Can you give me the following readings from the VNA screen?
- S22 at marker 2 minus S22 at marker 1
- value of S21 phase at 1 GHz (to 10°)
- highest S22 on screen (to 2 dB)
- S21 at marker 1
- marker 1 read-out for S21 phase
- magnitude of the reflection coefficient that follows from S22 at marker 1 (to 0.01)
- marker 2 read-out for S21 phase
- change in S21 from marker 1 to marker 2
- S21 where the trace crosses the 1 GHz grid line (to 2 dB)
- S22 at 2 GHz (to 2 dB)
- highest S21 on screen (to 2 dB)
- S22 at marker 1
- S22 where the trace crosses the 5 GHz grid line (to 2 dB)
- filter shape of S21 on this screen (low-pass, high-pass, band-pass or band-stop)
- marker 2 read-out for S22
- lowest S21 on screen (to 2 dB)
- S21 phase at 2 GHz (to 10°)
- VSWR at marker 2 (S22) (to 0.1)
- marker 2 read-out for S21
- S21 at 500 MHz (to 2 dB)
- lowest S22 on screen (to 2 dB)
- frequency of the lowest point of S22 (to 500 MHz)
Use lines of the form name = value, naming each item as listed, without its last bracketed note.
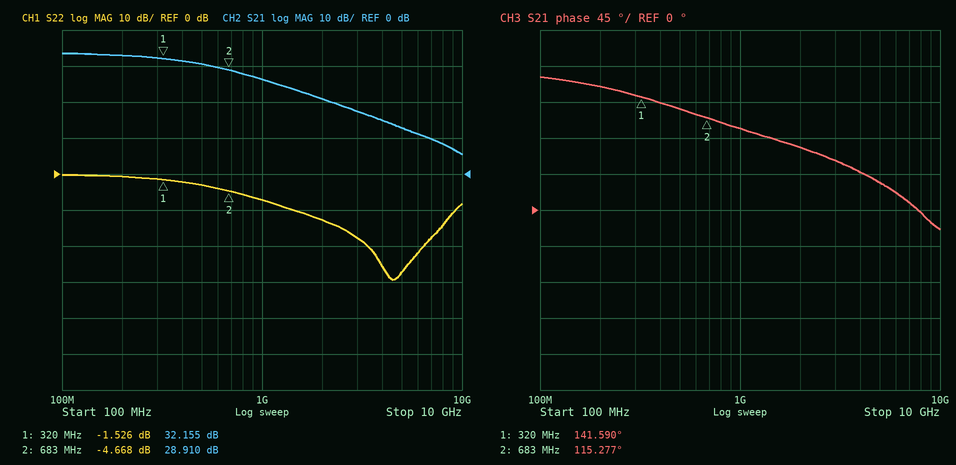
S22 at marker 2 minus S22 at marker 1 = -3.142 dB
value of S21 phase at 1 GHz = 100°
highest S22 on screen = 0 dB
S21 at marker 1 = 32.155 dB
marker 1 read-out for S21 phase = 141.590°
magnitude of the reflection coefficient that follows from S22 at marker 1 = 0.84
marker 2 read-out for S21 phase = 115.277°
change in S21 from marker 1 to marker 2 = -3.245 dB
S21 where the trace crosses the 1 GHz grid line = 26 dB
S22 at 2 GHz = -12 dB
highest S21 on screen = 34 dB
S22 at marker 1 = -1.526 dB
S22 where the trace crosses the 5 GHz grid line = -28 dB
filter shape of S21 on this screen = low-pass
marker 2 read-out for S22 = -4.668 dB
lowest S21 on screen = 6 dB
S21 phase at 2 GHz = 80°
VSWR at marker 2 (S22) = 3.8
marker 2 read-out for S21 = 28.910 dB
S21 at 500 MHz = 30 dB
lowest S22 on screen = -30 dB
frequency of the lowest point of S22 = 4.5 GHz
